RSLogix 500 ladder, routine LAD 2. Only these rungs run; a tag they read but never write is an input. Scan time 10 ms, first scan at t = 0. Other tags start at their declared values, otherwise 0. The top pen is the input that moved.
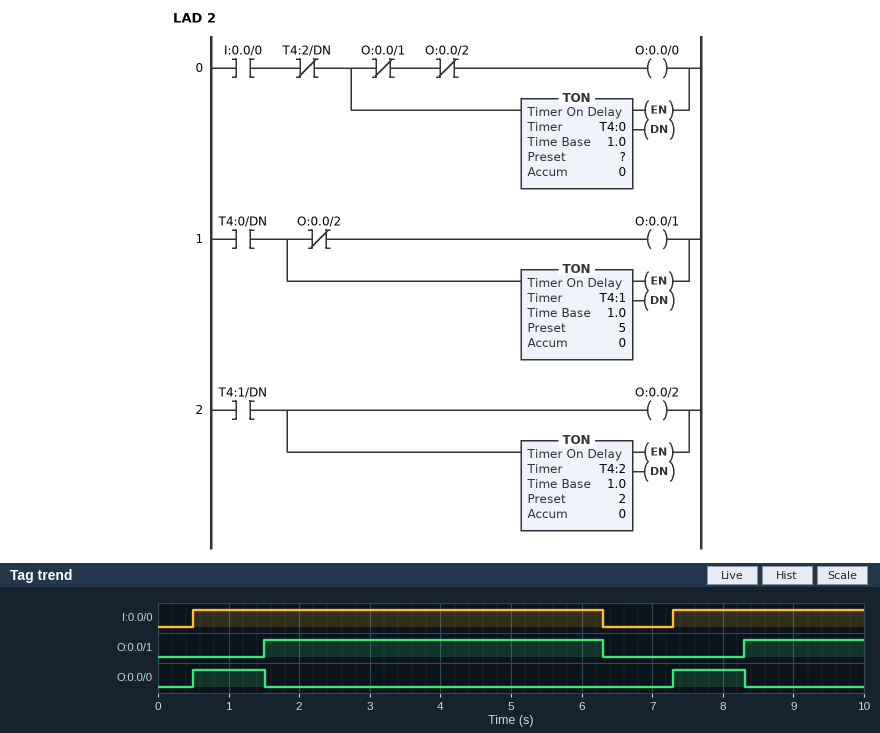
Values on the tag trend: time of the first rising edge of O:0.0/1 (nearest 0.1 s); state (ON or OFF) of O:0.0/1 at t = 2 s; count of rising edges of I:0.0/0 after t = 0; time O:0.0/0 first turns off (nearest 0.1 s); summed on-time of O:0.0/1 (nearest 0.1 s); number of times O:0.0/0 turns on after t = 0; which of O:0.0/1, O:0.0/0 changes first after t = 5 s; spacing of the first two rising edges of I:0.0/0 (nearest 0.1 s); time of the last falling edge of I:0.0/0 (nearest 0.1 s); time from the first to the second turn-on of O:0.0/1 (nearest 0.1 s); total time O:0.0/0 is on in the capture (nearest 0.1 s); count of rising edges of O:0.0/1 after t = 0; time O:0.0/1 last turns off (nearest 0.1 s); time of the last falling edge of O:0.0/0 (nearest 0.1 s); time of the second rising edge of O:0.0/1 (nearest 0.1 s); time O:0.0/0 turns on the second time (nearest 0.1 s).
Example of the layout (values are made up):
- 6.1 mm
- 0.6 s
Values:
- 1.5 s
- ON
- 2
- 1.5 s
- 6.5 s
- 2
- O:0.0/1
- 6.8 s
- 6.3 s
- 6.8 s
- 2.0 s
- 2
- 6.3 s
- 8.3 s
- 8.3 s
- 7.3 s
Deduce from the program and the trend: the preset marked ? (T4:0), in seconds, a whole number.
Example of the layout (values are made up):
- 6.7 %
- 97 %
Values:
- 1 s
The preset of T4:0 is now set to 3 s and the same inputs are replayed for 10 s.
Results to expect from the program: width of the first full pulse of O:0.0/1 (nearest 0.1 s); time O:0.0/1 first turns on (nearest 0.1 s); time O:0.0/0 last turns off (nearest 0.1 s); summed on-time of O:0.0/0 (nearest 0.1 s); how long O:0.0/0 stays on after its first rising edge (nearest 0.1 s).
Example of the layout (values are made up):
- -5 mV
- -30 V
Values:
- 2.8 s
- 3.5 s
- 3.5 s
- 5.7 s
- 3.0 s
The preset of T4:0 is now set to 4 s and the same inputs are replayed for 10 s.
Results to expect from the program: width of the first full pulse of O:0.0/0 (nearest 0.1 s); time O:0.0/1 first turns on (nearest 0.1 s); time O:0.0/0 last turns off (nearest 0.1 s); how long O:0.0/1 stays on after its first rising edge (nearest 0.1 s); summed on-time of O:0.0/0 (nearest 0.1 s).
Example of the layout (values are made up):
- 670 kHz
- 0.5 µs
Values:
- 4.0 s
- 4.5 s
- 4.5 s
- 1.8 s
- 6.7 s
